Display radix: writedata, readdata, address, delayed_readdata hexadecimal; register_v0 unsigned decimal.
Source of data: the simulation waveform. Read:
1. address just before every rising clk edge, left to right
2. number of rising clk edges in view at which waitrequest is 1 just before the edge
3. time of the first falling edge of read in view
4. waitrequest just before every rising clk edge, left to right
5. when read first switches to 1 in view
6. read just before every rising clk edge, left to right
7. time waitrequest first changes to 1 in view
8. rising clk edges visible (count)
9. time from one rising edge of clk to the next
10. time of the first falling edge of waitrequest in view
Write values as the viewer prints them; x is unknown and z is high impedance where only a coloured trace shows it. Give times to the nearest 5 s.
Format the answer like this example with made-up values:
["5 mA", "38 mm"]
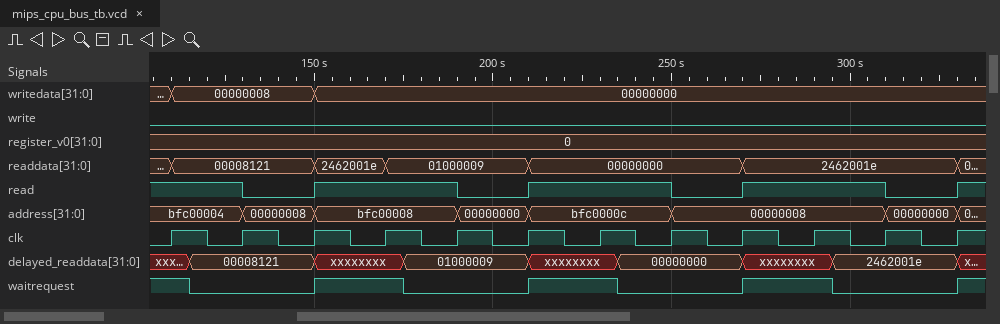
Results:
["bfc00004, bfc00004, 00000008, bfc00008, bfc00008, 00000000, bfc0000c, bfc0000c, 00000008, 00000008, 00000008, 00000000", "4", "130 s", "1 0 0 1 0 0 1 0 0 1 0 0", "150 s", "1 1 0 1 1 0 1 1 0 1 1 0", "150 s", "12", "20 s", "115 s"]
